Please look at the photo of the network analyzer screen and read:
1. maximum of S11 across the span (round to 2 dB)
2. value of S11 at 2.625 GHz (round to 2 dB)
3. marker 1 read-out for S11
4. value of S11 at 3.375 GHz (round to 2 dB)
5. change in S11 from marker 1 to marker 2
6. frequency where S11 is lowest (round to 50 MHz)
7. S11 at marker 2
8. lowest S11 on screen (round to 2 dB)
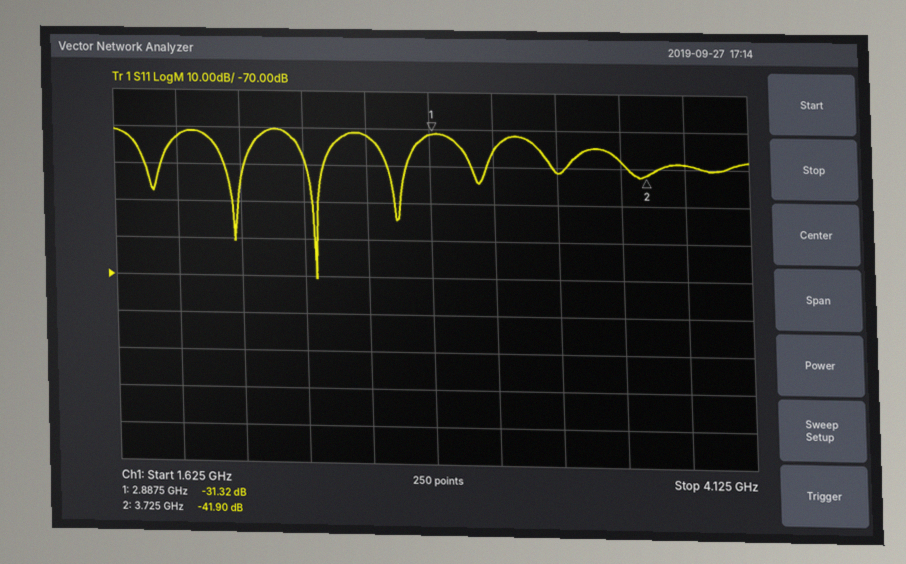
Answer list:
-30 dB
-32 dB
-31.32 dB
-42 dB
-10.58 dB
2.40 GHz
-41.90 dB
-70 dB
